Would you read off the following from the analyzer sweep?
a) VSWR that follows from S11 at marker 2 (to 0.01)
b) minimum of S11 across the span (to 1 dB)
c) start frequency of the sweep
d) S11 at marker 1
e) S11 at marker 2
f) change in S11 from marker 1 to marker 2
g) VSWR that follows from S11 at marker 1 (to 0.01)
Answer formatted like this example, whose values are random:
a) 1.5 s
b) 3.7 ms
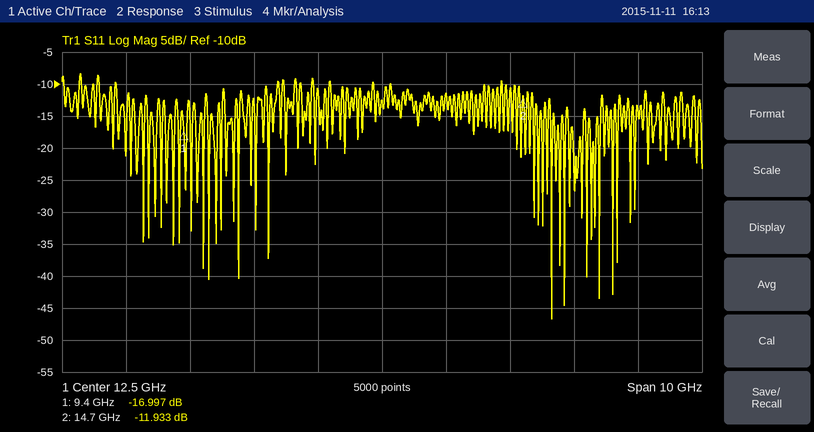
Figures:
a) 1.68
b) -47 dB
c) 7.5 GHz
d) -16.997 dB
e) -11.933 dB
f) 5.064 dB
g) 1.33
